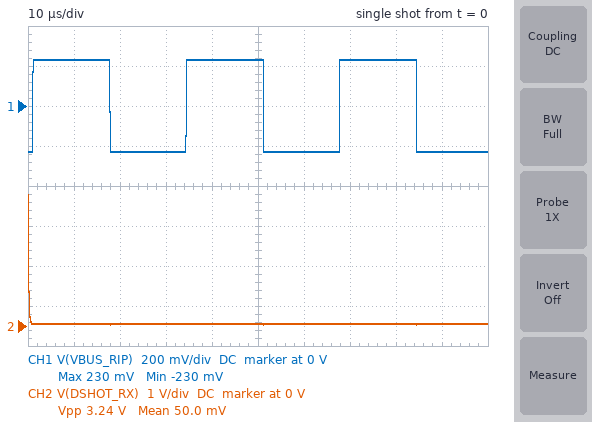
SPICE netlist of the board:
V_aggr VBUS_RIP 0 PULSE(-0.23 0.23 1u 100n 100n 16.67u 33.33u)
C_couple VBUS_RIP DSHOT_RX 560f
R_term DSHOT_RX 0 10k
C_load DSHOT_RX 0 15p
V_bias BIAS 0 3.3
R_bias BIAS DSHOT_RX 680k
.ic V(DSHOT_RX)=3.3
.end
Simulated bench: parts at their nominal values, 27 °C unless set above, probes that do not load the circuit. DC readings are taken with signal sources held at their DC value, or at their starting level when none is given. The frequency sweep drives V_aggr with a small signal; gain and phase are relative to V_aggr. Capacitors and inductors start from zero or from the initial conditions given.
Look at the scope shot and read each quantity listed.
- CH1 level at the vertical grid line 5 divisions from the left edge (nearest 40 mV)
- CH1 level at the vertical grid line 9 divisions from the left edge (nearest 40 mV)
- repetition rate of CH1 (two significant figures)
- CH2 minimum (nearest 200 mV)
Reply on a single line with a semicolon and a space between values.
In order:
240 mV; -240 mV; 30 kHz; 0 V
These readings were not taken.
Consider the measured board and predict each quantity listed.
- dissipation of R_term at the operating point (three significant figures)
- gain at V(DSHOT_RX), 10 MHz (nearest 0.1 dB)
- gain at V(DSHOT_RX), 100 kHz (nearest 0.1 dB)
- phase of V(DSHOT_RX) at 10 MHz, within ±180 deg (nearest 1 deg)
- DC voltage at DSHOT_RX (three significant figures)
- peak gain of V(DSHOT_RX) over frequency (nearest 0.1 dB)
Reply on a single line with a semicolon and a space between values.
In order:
229 nW; -28.9 dB; -49.2 dB; 6 deg; 47.8 mV; -28.9 dB
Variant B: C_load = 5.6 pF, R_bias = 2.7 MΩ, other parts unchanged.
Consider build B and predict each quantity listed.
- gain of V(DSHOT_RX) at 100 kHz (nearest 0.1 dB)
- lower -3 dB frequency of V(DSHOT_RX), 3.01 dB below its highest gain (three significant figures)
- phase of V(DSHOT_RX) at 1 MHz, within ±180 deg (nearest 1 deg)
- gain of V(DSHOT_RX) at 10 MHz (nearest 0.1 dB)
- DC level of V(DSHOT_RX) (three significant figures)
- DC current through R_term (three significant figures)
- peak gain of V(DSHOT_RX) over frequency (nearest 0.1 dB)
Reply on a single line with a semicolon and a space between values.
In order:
-49.1 dB; 2.59 MHz; 69 deg; -21.1 dB; 12.2 mV; 1.22 µA; -20.8 dB
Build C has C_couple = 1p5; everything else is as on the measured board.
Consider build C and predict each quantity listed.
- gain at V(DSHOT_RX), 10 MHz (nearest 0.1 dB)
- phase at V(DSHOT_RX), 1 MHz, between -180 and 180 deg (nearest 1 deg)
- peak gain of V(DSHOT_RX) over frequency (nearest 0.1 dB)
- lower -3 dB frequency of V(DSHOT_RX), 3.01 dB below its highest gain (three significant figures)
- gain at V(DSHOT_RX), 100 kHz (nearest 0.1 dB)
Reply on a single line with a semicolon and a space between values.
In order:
-20.9 dB; 44 deg; -20.8 dB; 979 kHz; -40.7 dB
